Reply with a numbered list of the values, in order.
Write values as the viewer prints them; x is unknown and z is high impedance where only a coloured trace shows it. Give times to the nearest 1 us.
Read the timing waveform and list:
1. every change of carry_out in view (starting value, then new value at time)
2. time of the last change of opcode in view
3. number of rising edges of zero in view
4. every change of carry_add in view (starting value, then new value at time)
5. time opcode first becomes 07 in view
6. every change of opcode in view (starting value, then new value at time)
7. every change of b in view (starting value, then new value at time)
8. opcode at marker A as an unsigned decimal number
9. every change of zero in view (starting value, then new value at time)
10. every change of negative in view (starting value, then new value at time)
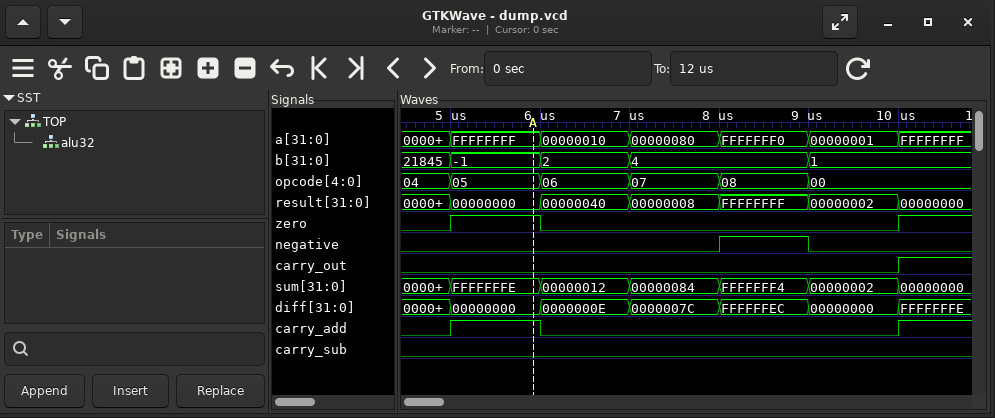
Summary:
1. 0, 1 at 10 us
2. 9 us
3. 2
4. 0, 1 at 5 us, 0 at 6 us, 1 at 10 us
5. 7 us
6. 04, 05 at 5 us, 06 at 6 us, 07 at 7 us, 08 at 8 us, 00 at 9 us
7. 21845, -1 at 5 us, 2 at 6 us, 4 at 7 us, 1 at 9 us
8. 5
9. 0, 1 at 5 us, 0 at 6 us, 1 at 10 us
10. 0, 1 at 8 us, 0 at 9 us
